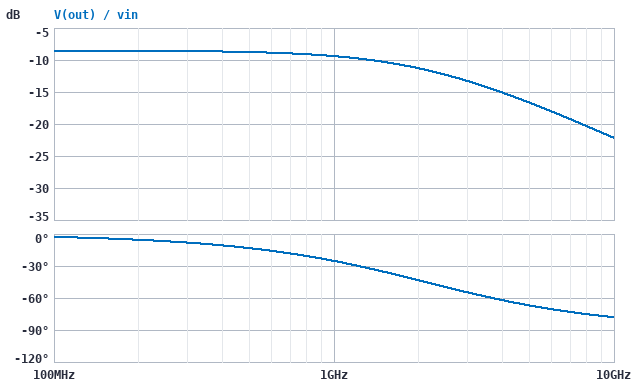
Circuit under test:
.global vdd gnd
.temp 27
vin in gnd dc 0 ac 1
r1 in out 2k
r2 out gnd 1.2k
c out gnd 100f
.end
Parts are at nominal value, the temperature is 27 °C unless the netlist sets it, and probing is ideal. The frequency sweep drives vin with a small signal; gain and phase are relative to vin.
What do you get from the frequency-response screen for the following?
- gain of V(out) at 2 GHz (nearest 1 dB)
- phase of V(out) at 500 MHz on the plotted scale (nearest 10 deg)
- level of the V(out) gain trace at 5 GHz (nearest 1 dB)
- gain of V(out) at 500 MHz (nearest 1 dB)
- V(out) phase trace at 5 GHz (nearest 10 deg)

-11 dB
-10 deg
-17 dB
-9 dB
-70 deg
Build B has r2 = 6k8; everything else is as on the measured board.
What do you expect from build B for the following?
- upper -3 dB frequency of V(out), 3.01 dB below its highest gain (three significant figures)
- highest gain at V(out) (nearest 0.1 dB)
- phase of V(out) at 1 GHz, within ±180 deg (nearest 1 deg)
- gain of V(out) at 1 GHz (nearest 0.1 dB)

1.03 GHz
-2.2 dB
-44 deg
-5.1 dB
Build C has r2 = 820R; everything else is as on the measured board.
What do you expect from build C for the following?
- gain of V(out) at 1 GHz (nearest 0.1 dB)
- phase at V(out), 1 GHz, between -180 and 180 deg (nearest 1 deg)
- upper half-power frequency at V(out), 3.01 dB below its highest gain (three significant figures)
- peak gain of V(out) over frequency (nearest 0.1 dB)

-11.3 dB
-20 deg
2.74 GHz
-10.7 dB
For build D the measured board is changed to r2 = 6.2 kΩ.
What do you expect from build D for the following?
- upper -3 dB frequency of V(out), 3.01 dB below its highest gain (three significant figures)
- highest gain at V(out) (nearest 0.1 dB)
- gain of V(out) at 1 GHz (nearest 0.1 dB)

1.05 GHz
-2.4 dB
-5.2 dB
